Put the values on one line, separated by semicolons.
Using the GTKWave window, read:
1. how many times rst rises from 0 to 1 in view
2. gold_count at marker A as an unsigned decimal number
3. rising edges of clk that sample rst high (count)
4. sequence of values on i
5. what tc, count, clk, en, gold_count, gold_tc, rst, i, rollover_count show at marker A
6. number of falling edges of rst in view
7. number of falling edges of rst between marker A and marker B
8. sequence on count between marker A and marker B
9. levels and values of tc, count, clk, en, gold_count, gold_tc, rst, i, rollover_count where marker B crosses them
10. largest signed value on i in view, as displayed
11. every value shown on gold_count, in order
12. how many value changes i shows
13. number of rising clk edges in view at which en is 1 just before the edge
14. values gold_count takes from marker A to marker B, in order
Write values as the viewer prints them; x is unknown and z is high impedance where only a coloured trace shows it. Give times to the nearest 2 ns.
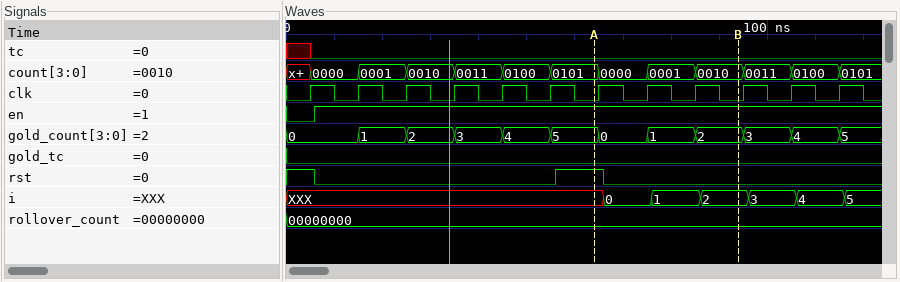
1; 5; 2; XXX, 0, 1, 2, 3, 4, 5; tc=0, count=0101, clk=0, en=1, gold_count=5, gold_tc=0, rst=1, i=XXX, rollover_count=00000000; 2; 1; 0101, 0000, 0001, 0010; tc=0, count=0010, clk=0, en=1, gold_count=2, gold_tc=0, rst=0, i=2, rollover_count=00000000; 5; 0, 1, 2, 3, 4, 5, 0, 1, 2, 3, 4, 5; 6; 11; 5, 0, 1, 2
